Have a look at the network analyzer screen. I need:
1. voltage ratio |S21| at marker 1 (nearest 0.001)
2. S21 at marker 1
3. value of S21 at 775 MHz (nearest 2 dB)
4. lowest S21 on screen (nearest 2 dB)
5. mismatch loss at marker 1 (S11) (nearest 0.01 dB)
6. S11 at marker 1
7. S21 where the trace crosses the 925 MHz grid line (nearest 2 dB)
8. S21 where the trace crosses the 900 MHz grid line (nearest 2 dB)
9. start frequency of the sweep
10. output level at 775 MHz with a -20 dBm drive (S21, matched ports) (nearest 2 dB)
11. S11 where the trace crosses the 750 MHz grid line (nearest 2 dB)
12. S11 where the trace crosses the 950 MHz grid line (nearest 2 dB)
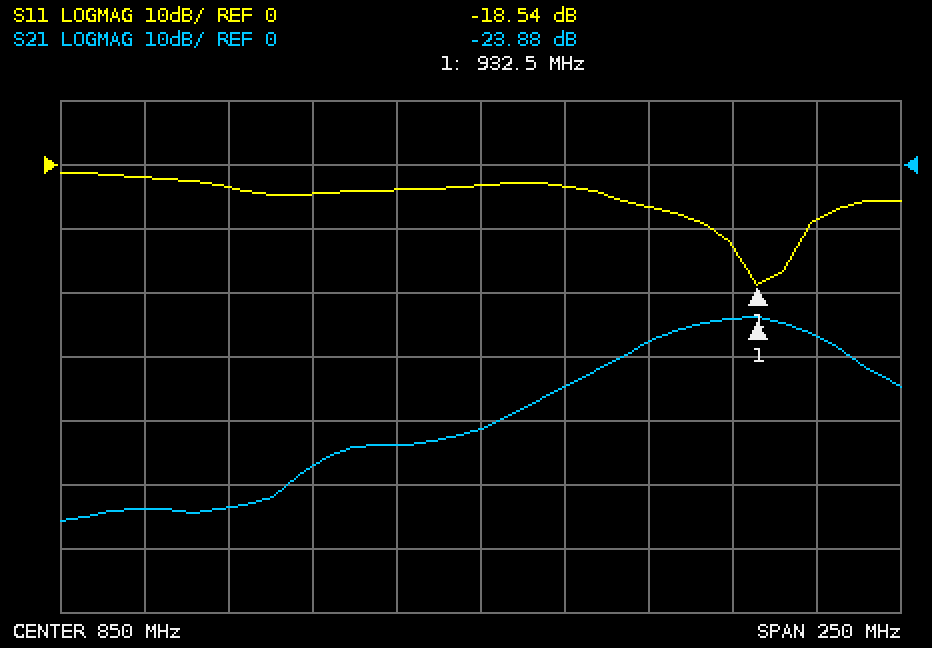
0.064
-23.88 dB
-54 dB
-56 dB
0.06 dB
-18.54 dB
-24 dB
-28 dB
725 MHz
-74 dBm
-2 dB
-8 dB
